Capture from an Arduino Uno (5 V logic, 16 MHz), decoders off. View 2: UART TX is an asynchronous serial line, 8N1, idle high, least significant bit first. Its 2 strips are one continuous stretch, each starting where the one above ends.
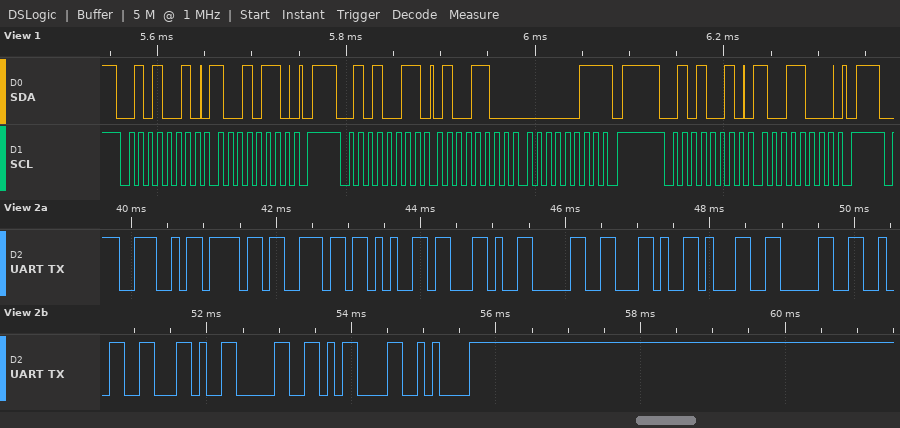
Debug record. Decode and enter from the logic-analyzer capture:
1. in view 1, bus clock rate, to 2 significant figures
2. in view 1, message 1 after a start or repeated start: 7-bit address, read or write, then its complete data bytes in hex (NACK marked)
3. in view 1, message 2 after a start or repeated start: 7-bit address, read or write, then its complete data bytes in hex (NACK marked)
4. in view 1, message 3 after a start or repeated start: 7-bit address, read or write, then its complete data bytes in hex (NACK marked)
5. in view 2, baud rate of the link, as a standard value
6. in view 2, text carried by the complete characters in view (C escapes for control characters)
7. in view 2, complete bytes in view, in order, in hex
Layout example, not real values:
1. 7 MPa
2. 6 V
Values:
1. 100 kHz
2. 0x29 write: 96
3. 0x29 read: 4C 03 NACK
4. 0x29 write: 98
5. 9600 baud
6. "None,0,102,0\r\n"
7. 0x4E 0x6F 0x6E 0x65 0x2C 0x30 0x2C 0x31 0x30 0x32 0x2C 0x30 0x0D 0x0A
